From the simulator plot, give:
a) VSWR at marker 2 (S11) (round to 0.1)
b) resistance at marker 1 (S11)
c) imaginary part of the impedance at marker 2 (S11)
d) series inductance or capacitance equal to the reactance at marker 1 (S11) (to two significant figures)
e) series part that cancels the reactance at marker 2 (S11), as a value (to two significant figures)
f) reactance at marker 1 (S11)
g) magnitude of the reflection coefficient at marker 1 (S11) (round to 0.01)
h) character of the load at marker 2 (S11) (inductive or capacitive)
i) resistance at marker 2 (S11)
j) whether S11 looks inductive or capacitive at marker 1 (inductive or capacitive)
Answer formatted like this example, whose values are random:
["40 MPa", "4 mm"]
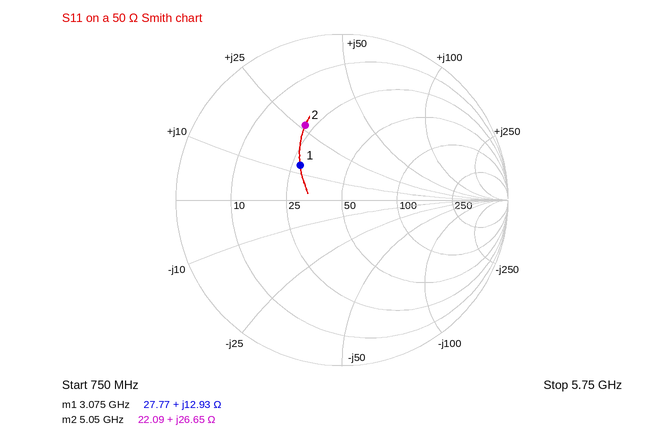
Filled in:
["3.0", "27.77 Ω", "+26.65 Ω", "670 pH", "1.2 pF", "+12.93 Ω", "0.33", "inductive", "22.09 Ω", "inductive"]
